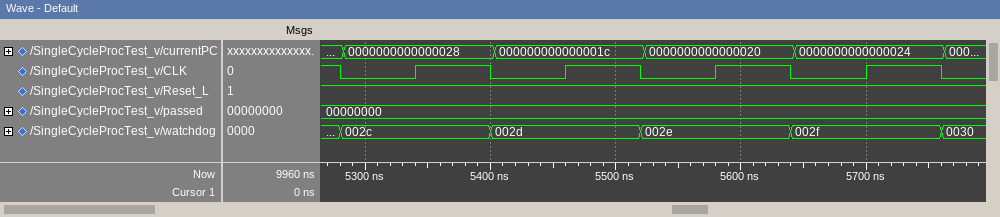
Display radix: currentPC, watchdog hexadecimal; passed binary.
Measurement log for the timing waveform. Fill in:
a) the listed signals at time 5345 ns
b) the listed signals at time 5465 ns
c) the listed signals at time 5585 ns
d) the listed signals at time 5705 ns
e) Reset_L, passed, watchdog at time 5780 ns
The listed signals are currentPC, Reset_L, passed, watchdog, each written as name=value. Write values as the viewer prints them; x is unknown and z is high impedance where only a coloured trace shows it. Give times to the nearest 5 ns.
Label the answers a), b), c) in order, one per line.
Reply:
a) currentPC=0000000000000028, Reset_L=1, passed=00000000, watchdog=002c
b) currentPC=000000000000001c, Reset_L=1, passed=00000000, watchdog=002d
c) currentPC=0000000000000020, Reset_L=1, passed=00000000, watchdog=002e
d) currentPC=0000000000000024, Reset_L=1, passed=00000000, watchdog=002f
e) Reset_L=1, passed=00000000, watchdog=0030
